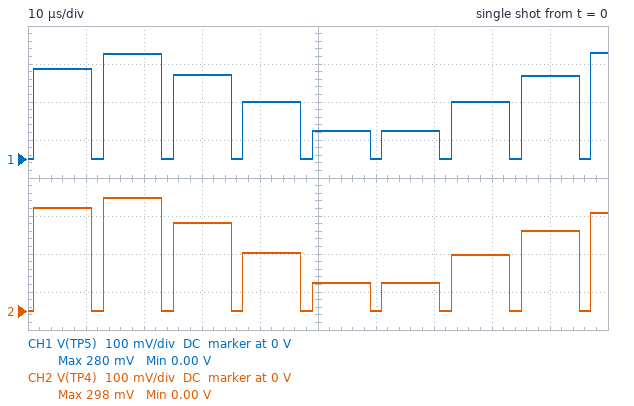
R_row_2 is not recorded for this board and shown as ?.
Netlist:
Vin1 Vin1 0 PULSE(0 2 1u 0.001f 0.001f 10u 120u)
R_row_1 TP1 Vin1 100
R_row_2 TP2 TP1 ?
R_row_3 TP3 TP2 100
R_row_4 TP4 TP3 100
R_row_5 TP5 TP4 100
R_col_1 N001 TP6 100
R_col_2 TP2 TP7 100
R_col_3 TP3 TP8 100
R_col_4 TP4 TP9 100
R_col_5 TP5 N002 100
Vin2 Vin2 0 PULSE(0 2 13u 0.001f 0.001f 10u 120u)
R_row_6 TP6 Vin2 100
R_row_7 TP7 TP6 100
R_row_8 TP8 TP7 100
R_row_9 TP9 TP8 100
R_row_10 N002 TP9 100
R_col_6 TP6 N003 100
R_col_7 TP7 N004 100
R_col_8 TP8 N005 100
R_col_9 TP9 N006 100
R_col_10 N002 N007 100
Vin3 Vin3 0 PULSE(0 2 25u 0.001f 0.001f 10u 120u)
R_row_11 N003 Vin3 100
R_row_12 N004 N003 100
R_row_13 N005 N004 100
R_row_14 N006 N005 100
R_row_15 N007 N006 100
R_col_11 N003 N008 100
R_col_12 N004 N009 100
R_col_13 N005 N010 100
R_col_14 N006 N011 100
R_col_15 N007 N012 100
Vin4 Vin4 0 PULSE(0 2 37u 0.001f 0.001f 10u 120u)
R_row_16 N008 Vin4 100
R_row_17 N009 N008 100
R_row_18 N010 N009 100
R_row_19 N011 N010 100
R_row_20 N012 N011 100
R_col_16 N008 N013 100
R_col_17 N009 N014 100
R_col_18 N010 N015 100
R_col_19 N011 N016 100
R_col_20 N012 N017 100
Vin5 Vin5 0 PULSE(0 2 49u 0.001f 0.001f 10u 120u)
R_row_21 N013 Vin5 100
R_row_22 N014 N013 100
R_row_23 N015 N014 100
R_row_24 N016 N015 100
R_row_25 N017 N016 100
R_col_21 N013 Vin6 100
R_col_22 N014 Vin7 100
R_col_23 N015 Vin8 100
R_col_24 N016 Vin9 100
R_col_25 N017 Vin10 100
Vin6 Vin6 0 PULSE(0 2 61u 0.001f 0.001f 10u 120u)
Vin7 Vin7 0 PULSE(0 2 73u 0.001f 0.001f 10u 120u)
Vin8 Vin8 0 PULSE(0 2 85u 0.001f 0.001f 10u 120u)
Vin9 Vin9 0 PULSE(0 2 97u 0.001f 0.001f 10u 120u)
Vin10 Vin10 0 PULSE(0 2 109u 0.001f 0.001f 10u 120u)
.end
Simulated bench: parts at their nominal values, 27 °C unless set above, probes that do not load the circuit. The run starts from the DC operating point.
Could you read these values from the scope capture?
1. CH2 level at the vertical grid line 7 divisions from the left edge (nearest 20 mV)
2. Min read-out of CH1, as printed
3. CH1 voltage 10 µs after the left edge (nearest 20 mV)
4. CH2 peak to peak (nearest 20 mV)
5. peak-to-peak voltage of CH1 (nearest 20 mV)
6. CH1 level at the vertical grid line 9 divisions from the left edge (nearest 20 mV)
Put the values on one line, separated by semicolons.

80 mV; 0.00 V; 240 mV; 300 mV; 280 mV; 220 mV
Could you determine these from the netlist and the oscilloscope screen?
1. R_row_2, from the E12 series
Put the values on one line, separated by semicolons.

220 Ω
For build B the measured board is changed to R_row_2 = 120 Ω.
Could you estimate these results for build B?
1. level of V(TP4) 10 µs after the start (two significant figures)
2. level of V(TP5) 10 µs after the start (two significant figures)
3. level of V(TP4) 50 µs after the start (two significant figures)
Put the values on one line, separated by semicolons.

350 mV; 310 mV; 71 mV
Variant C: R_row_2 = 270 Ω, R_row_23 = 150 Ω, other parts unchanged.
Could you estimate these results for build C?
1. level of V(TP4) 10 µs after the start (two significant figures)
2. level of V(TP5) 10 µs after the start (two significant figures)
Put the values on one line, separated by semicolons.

240 mV; 210 mV
